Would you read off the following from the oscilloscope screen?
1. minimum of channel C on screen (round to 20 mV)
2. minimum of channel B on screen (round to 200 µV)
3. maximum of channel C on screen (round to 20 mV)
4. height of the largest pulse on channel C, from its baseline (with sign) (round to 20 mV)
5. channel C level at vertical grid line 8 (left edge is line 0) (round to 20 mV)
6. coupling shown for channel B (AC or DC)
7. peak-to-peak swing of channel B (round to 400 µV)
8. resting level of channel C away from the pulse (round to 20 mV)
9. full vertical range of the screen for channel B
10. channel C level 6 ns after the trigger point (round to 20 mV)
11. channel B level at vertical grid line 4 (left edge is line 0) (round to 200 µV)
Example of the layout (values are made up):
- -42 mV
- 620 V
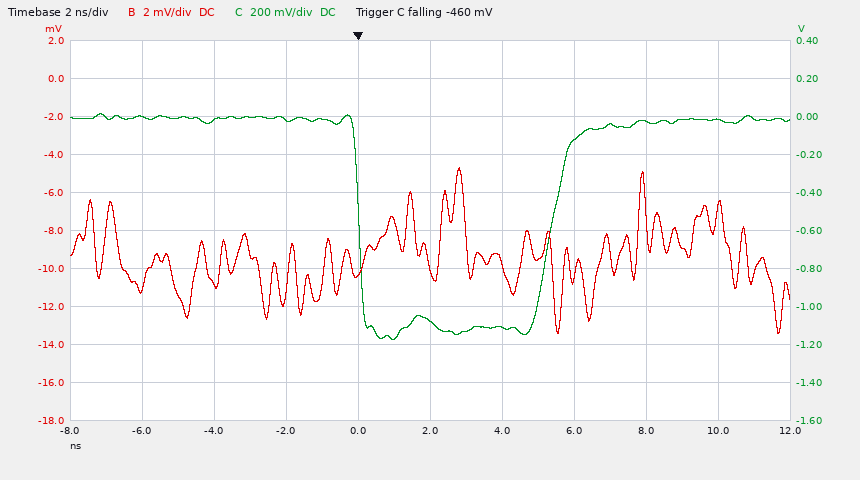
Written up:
- -1.18 V
- -13.4 mV
- 20 mV
- -1.16 V
- -20 mV
- DC
- 8.8 mV
- -20 mV
- 20 mV
- -120 mV
- -10.2 mV
